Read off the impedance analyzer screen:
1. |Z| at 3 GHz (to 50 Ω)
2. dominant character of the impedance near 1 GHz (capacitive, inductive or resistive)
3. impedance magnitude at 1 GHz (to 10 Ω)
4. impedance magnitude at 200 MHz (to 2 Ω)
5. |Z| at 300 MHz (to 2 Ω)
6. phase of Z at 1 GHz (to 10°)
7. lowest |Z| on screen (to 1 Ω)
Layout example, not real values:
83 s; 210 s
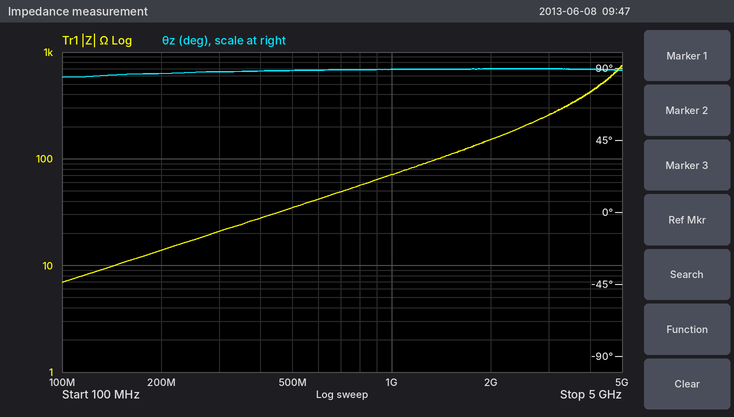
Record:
250 Ω; inductive; 70 Ω; 14 Ω; 20 Ω; 90°; 7 Ω
